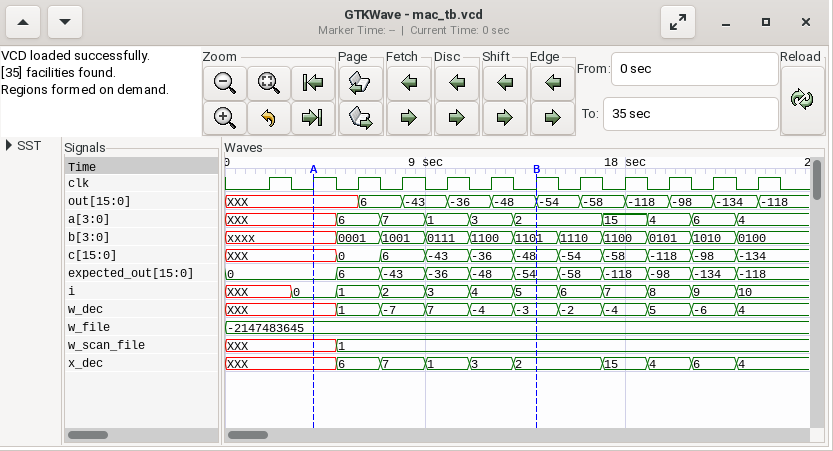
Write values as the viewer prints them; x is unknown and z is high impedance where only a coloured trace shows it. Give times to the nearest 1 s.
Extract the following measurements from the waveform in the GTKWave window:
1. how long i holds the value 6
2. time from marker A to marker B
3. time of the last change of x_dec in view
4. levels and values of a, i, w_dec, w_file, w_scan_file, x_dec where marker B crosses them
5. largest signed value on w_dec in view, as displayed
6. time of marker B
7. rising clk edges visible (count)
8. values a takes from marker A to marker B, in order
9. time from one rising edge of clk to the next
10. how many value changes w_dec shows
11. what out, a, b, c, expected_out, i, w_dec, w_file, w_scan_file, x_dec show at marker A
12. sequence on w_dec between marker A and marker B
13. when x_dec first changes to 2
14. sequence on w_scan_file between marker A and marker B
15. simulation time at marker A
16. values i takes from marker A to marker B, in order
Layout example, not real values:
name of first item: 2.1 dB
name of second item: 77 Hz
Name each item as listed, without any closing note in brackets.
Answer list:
how long i holds the value 6: 2 s
time from marker A to marker B: 10 s
time of the last change of x_dec in view: 23 s
levels and values of a, i, w_dec, w_file, w_scan_file, x_dec where marker B crosses them: a=2, i=5, w_dec=-3, w_file=-2147483645, w_scan_file=1, x_dec=2
largest signed value on w_dec in view, as displayed: 7
time of marker B: 14 s
rising clk edges visible: 12
values a takes from marker A to marker B, in order: XXX, 6, 7, 1, 3, 2
time from one rising edge of clk to the next: 2 s
how many value changes w_dec shows: 10
what out, a, b, c, expected_out, i, w_dec, w_file, w_scan_file, x_dec show at marker A: out=XXX, a=XXX, b=xxxx, c=XXX, expected_out=0, i=0, w_dec=XXX, w_file=-2147483645, w_scan_file=XXX, x_dec=XXX
sequence on w_dec between marker A and marker B: XXX, 1, -7, 7, -4, -3
when x_dec first changes to 2: 13 s
sequence on w_scan_file between marker A and marker B: XXX, 1
simulation time at marker A: 4 s
values i takes from marker A to marker B, in order: 0, 1, 2, 3, 4, 5
